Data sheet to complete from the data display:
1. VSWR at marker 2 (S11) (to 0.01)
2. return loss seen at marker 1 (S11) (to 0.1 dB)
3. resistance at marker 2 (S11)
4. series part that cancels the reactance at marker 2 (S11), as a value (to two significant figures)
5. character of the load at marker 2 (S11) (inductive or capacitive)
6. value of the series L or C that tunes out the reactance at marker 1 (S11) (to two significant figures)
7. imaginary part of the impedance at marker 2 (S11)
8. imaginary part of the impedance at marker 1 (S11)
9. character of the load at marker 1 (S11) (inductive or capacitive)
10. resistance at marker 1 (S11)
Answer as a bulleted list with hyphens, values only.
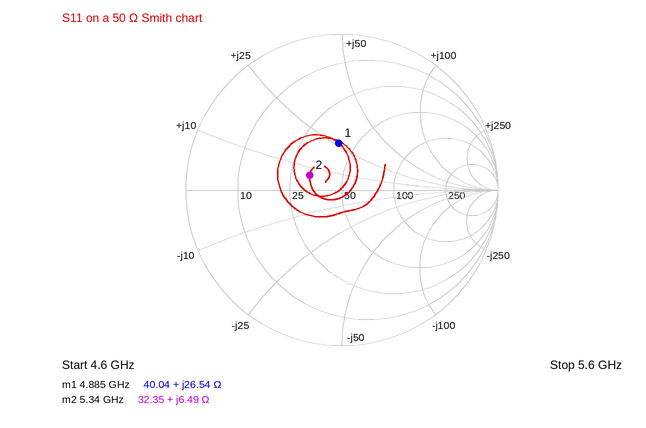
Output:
- 1.59
- 10.4 dB
- 32.35 Ω
- 4.6 pF
- inductive
- 1.2 pF
- +6.49 Ω
- +26.54 Ω
- inductive
- 40.04 Ω
